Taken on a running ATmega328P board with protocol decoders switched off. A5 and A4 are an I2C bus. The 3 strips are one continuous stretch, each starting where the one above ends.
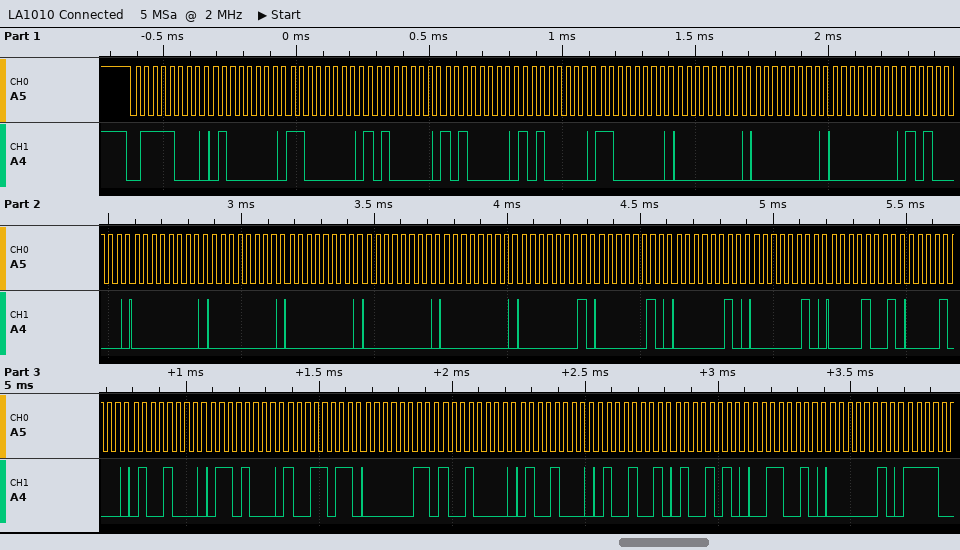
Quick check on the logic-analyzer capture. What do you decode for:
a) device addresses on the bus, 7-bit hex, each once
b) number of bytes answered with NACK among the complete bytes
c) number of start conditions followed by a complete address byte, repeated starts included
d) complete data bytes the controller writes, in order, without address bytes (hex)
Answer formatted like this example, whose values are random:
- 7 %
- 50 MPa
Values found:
- 0x3C
- 0
- 1
- 40 C0 A0 A0 A0 C0 00 00 00 A0 00 00 00 00 00 01 02 02 02 09 08 48 68 9B 03 90 48 49 4A 32 02
